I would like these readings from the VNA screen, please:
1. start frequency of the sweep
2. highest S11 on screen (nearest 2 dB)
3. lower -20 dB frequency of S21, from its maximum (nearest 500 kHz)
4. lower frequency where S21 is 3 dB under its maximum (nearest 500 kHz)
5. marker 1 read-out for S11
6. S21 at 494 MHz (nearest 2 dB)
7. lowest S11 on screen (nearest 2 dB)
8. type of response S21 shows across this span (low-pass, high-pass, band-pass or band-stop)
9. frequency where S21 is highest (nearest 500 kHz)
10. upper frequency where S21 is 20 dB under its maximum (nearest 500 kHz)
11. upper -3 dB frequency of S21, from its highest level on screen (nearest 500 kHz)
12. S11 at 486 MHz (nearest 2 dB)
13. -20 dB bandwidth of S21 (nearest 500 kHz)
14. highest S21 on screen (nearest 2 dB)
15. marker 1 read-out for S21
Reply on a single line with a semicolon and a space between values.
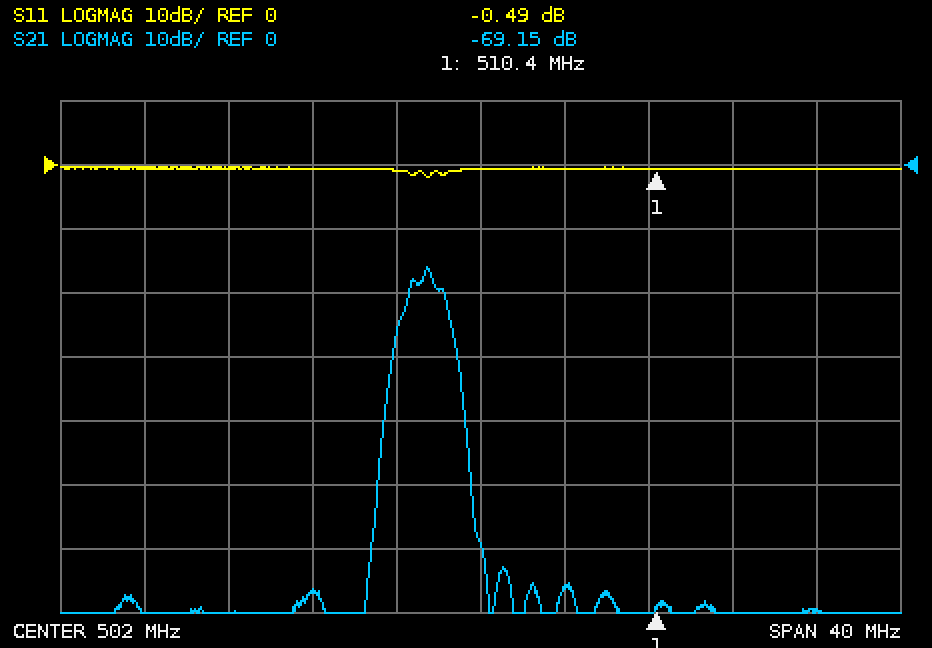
482 MHz; 0 dB; 497.5 MHz; 498.5 MHz; -0.49 dB; -66 dB; -2 dB; band-pass; 499.5 MHz; 501.0 MHz; 500.0 MHz; 0 dB; 3.5 MHz; -16 dB; -69.15 dB
